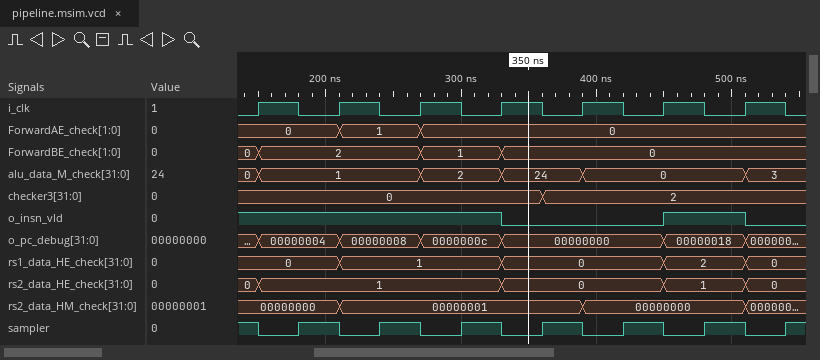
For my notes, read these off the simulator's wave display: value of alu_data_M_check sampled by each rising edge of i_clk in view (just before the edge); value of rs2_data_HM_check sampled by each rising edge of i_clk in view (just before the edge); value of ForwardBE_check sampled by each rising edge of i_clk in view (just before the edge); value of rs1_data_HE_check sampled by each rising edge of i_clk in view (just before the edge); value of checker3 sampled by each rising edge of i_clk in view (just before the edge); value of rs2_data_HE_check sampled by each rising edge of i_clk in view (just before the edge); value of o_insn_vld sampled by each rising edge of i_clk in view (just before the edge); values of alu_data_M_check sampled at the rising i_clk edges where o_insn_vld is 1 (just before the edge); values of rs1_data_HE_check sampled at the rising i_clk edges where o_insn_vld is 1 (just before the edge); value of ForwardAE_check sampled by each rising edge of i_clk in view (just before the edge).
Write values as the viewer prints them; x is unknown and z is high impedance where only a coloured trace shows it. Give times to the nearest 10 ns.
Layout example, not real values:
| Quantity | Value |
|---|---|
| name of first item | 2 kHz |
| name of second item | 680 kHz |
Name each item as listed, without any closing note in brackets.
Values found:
| Quantity | Value |
|---|---|
| value of alu_data_M_check sampled by each rising edge of i_clk in view | 0, 1, 1, 2, 24, 0, 0 |
| value of rs2_data_HM_check sampled by each rising edge of i_clk in view | 00000000, 00000000, 00000001, 00000001, 00000001, 00000000, 00000000 |
| value of ForwardBE_check sampled by each rising edge of i_clk in view | 0, 2, 2, 1, 0, 0, 0 |
| value of rs1_data_HE_check sampled by each rising edge of i_clk in view | 0, 0, 1, 1, 0, 0, 2 |
| value of checker3 sampled by each rising edge of i_clk in view | 0, 0, 0, 0, 2, 2, 2 |
| value of rs2_data_HE_check sampled by each rising edge of i_clk in view | 0, 1, 1, 1, 0, 0, 1 |
| value of o_insn_vld sampled by each rising edge of i_clk in view | 1 1 1 1 0 0 1 |
| values of alu_data_M_check sampled at the rising i_clk edges where o_insn_vld is 1 | 0, 1, 1, 2, 0 |
| values of rs1_data_HE_check sampled at the rising i_clk edges where o_insn_vld is 1 | 0, 0, 1, 1, 2 |
| value of ForwardAE_check sampled by each rising edge of i_clk in view | 0, 0, 1, 0, 0, 0, 0 |
